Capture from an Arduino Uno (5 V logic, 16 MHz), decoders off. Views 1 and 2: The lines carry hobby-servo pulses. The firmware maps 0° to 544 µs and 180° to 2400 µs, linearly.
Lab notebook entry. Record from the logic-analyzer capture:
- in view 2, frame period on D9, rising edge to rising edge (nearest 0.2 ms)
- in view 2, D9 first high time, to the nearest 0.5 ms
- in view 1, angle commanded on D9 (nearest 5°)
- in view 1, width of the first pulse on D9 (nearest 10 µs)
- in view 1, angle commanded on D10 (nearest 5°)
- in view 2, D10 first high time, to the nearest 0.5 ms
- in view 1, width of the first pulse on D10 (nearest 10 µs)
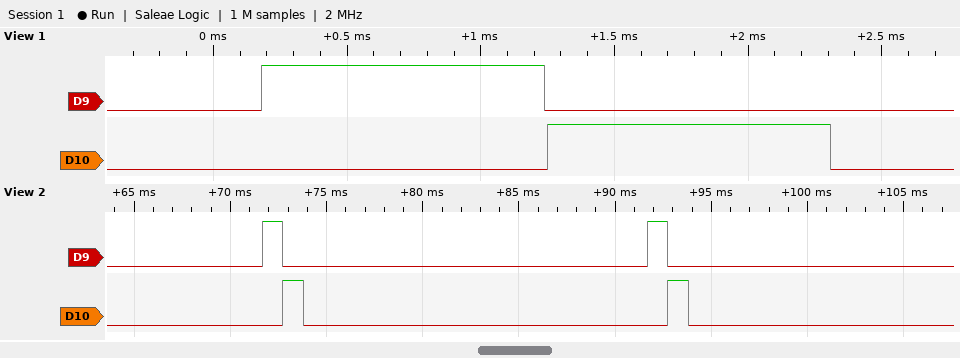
20.0 ms
1.0 ms
50°
1060 µs
50°
1.0 ms
1060 µs
